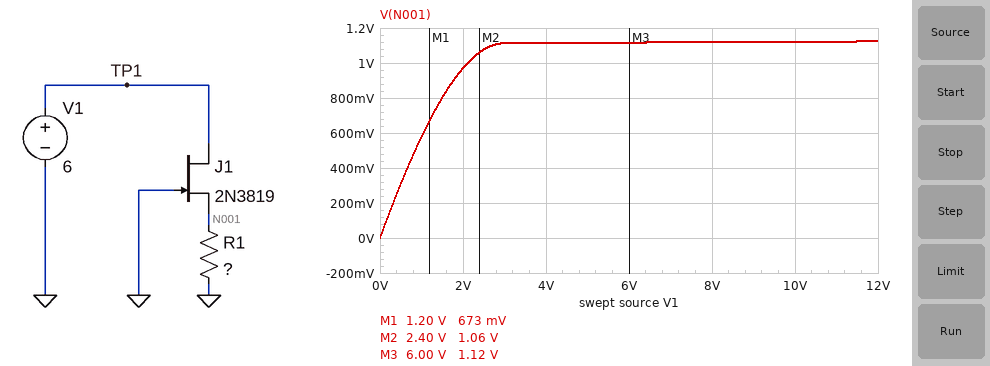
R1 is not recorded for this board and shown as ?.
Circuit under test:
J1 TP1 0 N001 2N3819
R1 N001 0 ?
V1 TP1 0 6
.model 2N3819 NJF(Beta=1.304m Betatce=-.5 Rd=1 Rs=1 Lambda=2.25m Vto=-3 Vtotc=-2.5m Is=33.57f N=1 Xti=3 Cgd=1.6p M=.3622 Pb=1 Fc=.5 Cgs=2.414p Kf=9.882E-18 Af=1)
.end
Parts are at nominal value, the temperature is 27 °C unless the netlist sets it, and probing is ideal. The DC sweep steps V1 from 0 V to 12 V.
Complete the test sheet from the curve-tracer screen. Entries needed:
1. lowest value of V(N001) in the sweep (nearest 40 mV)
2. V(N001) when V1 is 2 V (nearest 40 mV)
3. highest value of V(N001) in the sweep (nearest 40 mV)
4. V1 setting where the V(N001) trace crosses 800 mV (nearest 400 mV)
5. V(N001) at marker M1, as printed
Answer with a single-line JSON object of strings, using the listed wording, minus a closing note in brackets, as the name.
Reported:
{"lowest value of V(N001) in the sweep": "0 V", "V(N001) when V1 is 2 V": "960 mV", "highest value of V(N001) in the sweep": "1.12 V", "V1 setting where the V(N001) trace crosses 800 mV": "1.6 V", "V(N001) at marker M1, as printed": "673 mV"}
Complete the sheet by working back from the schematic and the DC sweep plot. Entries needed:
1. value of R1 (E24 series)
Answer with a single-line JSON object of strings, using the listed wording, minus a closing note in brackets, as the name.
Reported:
{"value of R1": "240 Ω"}
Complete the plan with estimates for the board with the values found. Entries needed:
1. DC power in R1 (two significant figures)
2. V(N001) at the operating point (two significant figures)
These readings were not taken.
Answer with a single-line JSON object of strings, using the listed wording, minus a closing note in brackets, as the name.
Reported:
{"DC power in R1": "5.2 mW", "V(N001) at the operating point": "1.1 V"}
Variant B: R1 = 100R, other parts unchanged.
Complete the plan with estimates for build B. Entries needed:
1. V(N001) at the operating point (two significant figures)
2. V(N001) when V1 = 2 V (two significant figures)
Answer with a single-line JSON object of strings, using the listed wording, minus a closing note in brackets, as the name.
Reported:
{"V(N001) at the operating point": "700 mV", "V(N001) when V1 = 2 V": "610 mV"}
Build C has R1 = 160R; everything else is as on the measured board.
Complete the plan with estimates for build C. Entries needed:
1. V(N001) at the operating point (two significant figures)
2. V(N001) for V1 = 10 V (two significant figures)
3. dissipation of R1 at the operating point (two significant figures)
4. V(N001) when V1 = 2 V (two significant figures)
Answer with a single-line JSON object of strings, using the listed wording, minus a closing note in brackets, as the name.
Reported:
{"V(N001) at the operating point": "910 mV", "V(N001) for V1 = 10 V": "920 mV", "dissipation of R1 at the operating point": "5.2 mW", "V(N001) when V1 = 2 V": "800 mV"}
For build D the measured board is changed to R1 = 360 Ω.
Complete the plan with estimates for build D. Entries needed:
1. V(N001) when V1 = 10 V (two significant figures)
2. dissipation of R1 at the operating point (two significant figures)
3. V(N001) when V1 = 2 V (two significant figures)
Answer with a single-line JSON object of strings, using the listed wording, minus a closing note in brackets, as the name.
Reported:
{"V(N001) when V1 = 10 V": "1.3 V", "dissipation of R1 at the operating point": "4.9 mW", "V(N001) when V1 = 2 V": "1.1 V"}
